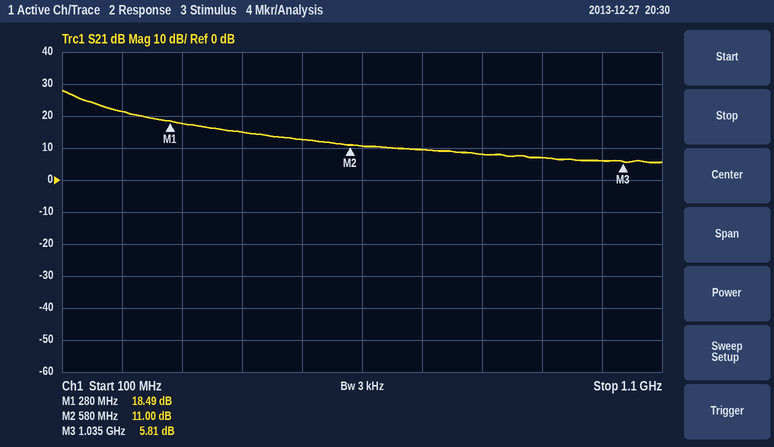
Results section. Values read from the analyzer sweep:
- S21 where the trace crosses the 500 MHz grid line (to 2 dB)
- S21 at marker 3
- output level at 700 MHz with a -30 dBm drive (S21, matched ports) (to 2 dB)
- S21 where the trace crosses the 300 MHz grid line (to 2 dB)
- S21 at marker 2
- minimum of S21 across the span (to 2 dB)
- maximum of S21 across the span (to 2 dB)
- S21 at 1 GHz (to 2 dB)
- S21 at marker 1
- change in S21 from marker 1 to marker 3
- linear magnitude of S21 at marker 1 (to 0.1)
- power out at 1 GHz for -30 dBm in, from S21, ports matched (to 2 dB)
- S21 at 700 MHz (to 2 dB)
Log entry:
12 dB
5.81 dB
-20 dBm
18 dB
11.00 dB
6 dB
28 dB
6 dB
18.49 dB
-12.68 dB
8.4
-24 dBm
10 dB
